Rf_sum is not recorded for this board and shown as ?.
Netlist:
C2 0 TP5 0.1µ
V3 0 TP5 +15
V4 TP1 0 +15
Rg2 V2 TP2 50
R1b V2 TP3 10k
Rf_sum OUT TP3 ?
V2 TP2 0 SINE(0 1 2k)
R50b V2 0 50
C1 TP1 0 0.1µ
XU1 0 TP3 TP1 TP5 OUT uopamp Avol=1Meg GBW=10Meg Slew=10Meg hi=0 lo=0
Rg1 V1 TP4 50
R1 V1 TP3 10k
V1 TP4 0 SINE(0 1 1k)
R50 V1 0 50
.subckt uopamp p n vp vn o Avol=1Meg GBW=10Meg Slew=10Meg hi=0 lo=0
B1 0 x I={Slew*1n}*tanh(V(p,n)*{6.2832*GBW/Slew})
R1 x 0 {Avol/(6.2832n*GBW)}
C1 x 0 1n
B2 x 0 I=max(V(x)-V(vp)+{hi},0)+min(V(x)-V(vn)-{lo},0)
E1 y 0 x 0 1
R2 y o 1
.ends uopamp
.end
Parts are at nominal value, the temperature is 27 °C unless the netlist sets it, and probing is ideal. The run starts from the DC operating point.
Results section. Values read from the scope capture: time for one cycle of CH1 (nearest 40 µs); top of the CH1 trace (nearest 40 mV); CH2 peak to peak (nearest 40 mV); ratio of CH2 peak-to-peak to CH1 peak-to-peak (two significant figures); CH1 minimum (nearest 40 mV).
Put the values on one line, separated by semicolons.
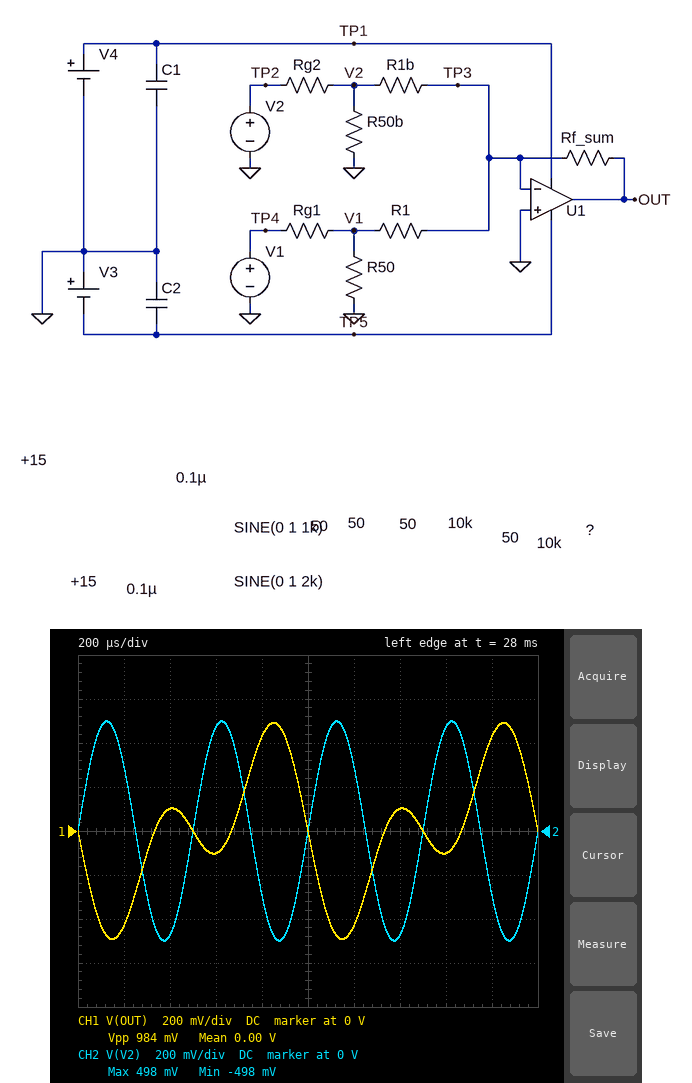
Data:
1.00 ms; 480 mV; 1.00 V; 1.0; -480 mV
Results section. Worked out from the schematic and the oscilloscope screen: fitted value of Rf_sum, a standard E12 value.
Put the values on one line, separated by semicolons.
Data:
5.6 kΩ
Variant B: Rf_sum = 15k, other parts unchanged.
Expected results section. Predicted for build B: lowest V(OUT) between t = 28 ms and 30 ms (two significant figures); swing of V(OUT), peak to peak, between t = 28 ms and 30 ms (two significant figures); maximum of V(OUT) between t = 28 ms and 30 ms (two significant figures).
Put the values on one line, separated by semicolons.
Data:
-1.3 V; 2.6 V; 1.3 V
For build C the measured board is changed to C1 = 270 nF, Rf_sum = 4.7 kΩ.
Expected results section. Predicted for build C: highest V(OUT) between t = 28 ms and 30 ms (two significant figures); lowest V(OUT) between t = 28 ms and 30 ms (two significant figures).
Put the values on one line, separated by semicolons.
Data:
410 mV; -410 mV
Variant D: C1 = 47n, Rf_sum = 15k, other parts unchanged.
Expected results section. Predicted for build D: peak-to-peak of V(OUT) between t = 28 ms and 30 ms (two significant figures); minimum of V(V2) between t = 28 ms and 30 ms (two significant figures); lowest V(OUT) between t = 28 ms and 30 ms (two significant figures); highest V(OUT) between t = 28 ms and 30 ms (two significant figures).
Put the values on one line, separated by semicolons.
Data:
2.6 V; -500 mV; -1.3 V; 1.3 V
